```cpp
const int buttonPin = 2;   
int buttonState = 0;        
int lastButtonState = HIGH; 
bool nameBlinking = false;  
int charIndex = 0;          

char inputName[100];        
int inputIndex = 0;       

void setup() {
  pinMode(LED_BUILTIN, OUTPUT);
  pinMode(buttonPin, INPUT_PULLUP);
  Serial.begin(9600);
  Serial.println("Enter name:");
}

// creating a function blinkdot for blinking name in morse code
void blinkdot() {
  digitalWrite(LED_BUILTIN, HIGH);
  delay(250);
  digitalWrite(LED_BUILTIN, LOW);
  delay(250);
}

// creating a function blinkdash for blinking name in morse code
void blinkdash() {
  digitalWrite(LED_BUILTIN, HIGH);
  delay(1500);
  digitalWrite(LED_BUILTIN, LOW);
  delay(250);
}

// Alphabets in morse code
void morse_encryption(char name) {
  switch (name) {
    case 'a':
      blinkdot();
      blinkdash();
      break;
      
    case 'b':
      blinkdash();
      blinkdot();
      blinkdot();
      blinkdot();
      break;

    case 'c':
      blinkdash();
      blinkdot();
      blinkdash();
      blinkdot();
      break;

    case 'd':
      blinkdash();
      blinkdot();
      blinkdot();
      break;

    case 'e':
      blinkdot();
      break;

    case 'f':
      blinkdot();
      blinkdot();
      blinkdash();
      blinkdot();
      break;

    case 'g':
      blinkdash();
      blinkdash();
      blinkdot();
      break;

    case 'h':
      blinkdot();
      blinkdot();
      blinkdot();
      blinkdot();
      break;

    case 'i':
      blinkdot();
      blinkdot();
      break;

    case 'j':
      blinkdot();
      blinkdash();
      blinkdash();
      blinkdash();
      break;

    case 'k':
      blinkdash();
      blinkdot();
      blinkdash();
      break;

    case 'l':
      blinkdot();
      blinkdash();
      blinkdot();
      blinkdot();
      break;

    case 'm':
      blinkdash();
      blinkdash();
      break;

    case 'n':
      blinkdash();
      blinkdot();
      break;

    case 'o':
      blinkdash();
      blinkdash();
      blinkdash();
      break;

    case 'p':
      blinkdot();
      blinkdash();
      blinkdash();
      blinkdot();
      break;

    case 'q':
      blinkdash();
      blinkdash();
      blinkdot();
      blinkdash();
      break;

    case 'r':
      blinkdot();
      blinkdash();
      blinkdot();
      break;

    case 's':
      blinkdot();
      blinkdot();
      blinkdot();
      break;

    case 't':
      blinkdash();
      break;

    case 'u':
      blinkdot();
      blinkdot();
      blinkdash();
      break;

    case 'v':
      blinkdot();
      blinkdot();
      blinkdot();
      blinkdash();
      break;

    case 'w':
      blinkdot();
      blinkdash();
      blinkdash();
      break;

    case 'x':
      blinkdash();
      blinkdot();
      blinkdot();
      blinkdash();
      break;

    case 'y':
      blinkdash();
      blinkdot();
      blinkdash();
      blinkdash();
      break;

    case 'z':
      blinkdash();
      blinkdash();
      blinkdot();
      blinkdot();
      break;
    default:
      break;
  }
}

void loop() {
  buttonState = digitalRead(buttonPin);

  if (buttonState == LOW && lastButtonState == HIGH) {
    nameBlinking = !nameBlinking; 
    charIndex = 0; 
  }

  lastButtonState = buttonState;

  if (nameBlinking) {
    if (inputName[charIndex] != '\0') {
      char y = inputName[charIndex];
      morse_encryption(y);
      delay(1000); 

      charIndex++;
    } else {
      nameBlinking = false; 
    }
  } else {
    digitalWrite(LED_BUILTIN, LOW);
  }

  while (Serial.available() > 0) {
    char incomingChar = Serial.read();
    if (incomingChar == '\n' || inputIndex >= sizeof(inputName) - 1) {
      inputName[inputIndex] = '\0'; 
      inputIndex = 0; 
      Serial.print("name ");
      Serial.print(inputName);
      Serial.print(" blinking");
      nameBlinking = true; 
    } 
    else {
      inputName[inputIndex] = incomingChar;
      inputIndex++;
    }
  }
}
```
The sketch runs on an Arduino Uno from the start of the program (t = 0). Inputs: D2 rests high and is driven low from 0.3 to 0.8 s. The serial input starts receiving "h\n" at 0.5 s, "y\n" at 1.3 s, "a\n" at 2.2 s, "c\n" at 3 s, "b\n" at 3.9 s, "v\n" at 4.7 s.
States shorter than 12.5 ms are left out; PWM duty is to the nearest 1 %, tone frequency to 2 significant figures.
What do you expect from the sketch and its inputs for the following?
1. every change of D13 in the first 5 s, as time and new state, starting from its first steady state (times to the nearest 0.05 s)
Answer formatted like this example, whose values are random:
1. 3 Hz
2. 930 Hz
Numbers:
1. 0 s low; 0.5 s high; 0.75 s low; 1 s high; 1.25 s low; 1.5 s high; 1.75 s low; 2 s high; 2.25 s low
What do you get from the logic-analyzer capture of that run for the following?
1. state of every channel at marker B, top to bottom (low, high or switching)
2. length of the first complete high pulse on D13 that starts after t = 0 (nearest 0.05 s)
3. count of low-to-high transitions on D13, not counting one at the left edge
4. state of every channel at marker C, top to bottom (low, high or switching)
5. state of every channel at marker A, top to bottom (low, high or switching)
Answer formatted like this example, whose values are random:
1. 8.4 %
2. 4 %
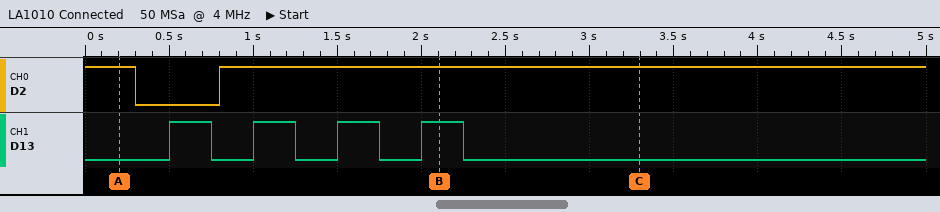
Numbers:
1. D2 high, D13 high
2. 0.25 s
3. 4
4. D2 high, D13 low
5. D2 high, D13 low
